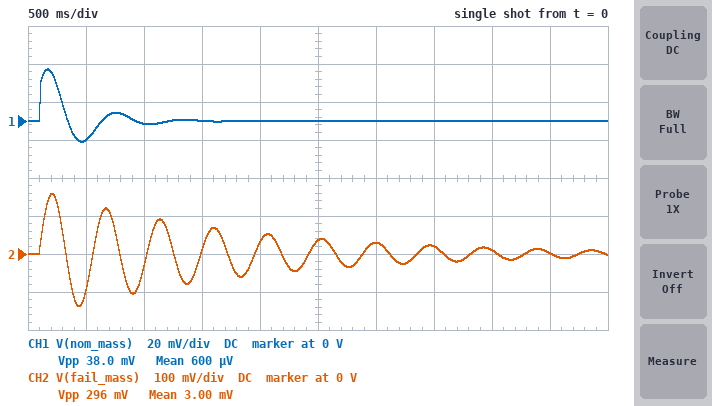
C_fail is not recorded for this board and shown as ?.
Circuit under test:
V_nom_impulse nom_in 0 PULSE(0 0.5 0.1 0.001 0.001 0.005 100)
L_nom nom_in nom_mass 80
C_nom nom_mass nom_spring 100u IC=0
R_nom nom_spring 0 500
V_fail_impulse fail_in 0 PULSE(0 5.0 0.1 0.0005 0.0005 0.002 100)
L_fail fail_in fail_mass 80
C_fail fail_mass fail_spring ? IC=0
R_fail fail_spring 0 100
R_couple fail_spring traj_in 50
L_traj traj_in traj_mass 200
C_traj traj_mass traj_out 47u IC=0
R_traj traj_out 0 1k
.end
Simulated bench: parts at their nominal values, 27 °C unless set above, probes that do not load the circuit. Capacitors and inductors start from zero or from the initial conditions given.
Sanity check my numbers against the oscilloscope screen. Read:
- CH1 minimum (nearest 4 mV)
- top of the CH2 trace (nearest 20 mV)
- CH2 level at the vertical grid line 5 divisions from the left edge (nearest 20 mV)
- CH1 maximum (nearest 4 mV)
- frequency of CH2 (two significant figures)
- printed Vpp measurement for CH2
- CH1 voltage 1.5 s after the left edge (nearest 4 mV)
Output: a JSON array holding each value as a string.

["-12 mV", "160 mV", "40 mV", "28 mV", "2.1 Hz", "296 mV", "0 V"]
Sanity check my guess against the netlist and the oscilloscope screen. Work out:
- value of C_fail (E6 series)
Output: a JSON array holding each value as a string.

["68 µF"]
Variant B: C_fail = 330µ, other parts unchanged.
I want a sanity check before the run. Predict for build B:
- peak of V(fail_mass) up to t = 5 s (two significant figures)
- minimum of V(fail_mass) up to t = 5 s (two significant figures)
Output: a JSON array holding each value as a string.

["68 mV", "-50 mV"]
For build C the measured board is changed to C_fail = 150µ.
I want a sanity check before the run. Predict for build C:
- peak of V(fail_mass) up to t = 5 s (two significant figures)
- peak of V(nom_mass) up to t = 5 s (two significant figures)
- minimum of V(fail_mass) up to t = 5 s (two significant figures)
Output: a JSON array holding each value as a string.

["100 mV", "27 mV", "-85 mV"]
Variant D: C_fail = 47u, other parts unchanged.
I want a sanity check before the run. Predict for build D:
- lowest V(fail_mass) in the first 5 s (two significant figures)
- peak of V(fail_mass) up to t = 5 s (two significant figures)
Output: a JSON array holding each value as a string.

["-170 mV", "190 mV"]
